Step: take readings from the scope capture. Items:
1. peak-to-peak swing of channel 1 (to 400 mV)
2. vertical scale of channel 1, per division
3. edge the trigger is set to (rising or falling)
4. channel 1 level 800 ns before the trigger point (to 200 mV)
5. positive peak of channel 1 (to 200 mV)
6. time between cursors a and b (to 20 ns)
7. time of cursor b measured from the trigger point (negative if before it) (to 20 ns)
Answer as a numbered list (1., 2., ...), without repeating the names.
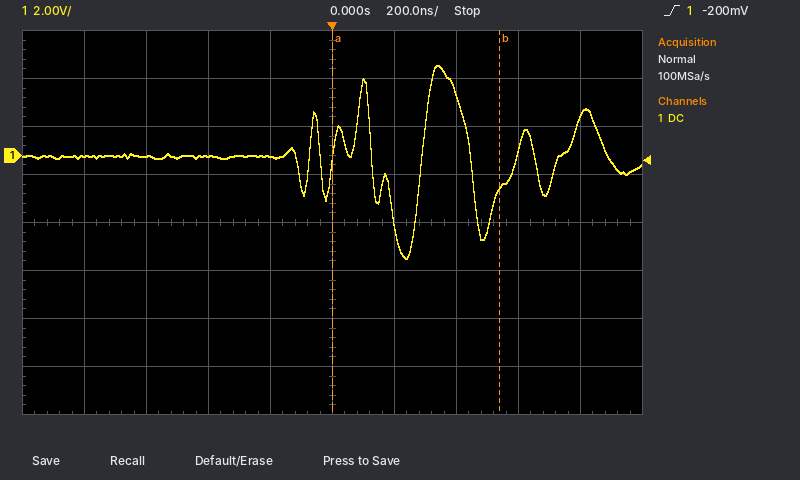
1. 8.0 V
2. 2 V
3. rising
4. 0.0 V
5. 3.8 V
6. 540 ns
7. +540 ns
